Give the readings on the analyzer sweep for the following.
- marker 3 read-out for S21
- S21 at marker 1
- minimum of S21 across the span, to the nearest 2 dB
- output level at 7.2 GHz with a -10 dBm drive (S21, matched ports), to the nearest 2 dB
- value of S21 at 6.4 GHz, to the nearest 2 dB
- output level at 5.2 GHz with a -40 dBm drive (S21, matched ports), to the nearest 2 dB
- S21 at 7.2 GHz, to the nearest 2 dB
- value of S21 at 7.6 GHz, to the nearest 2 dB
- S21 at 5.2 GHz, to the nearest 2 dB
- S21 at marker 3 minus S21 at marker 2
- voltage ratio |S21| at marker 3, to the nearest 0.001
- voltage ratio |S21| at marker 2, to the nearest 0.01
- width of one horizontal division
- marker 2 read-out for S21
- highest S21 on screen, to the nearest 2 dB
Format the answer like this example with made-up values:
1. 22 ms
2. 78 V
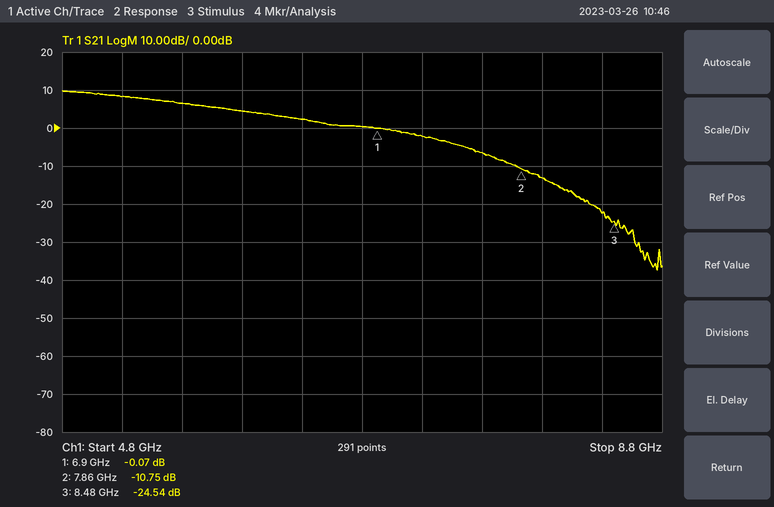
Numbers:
1. -24.54 dB
2. -0.07 dB
3. -38 dB
4. -12 dBm
5. 2 dB
6. -32 dBm
7. -2 dB
8. -6 dB
9. 8 dB
10. -13.79 dB
11. 0.059
12. 0.29
13. 400 MHz
14. -10.75 dB
15. 10 dB
